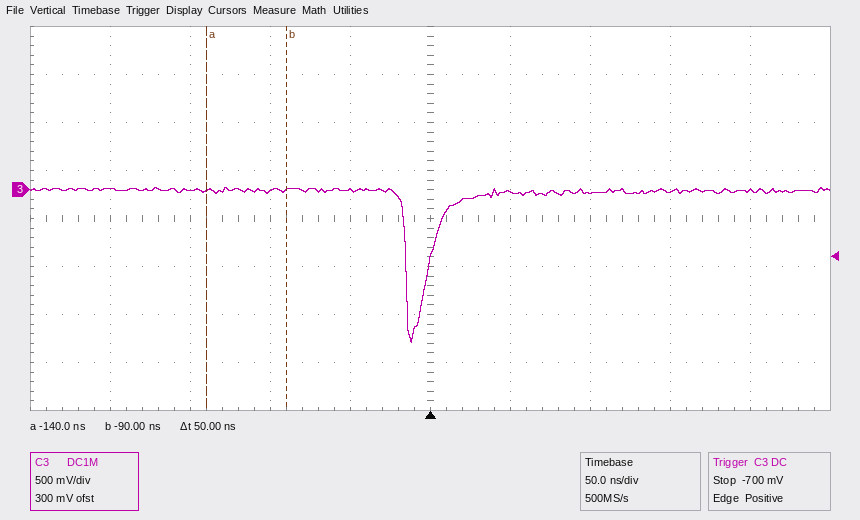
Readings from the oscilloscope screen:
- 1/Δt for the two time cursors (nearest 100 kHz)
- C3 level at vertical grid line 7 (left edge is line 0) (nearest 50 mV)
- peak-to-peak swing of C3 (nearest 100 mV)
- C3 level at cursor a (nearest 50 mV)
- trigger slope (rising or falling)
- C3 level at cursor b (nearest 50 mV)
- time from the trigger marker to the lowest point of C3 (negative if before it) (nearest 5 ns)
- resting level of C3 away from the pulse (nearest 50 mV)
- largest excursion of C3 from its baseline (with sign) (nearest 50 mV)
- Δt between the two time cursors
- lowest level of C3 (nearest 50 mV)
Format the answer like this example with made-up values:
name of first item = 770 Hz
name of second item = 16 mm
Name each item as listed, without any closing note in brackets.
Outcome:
1/Δt for the two time cursors = 20.0 MHz
C3 level at vertical grid line 7 (left edge is line 0) = -50 mV
peak-to-peak swing of C3 = 1.60 V
C3 level at cursor a = 0 mV
trigger slope = rising
C3 level at cursor b = 0 mV
time from the trigger marker to the lowest point of C3 (negative if before it) = -10 ns
resting level of C3 away from the pulse = 0 mV
largest excursion of C3 from its baseline (with sign) = -1.60 V
Δt between the two time cursors = 50 ns
lowest level of C3 = -1.60 V
